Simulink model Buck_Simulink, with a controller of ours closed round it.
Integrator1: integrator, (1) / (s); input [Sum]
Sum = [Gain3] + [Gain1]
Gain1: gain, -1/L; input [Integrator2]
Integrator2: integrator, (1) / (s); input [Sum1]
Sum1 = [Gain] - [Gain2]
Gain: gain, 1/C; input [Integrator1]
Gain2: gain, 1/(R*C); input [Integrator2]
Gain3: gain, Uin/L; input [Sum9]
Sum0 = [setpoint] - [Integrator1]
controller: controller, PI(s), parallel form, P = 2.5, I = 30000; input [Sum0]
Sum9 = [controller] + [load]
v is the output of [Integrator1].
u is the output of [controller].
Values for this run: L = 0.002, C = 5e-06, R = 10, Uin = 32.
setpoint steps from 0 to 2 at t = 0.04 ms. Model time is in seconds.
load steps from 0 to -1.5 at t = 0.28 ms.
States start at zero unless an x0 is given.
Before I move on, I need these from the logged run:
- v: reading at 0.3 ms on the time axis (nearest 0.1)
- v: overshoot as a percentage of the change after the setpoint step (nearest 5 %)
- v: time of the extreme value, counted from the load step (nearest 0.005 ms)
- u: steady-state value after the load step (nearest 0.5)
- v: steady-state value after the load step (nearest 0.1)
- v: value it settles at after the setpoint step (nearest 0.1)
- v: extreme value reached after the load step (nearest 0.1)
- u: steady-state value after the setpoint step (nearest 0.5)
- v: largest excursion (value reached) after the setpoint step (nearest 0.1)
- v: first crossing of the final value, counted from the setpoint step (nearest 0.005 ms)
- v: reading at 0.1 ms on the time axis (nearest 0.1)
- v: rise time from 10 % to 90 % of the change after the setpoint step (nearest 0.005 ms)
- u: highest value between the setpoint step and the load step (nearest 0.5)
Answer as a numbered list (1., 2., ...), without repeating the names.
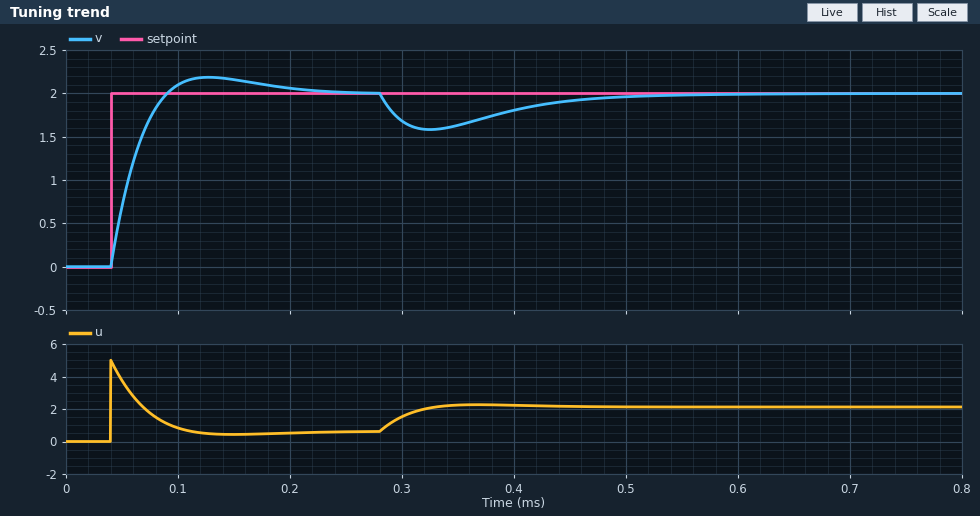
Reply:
1. 1.7
2. 10 %
3. 0.045 ms
4. 2.0
5. 2.0
6. 2.0
7. 1.6
8. 0.5
9. 2.2
10. 0.050 ms
11. 2.1
12. 0.035 ms
13. 5.0
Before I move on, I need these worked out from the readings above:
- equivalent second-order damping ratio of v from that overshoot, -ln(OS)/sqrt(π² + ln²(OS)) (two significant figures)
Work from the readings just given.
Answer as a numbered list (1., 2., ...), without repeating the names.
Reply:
1. 0.59
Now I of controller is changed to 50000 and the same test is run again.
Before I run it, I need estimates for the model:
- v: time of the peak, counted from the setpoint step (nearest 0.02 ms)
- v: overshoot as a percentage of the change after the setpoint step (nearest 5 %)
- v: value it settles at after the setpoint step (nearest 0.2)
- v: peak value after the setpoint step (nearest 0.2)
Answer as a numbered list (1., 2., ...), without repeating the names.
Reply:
1. 0.08 ms
2. 15 %
3. 2.0
4. 2.4
